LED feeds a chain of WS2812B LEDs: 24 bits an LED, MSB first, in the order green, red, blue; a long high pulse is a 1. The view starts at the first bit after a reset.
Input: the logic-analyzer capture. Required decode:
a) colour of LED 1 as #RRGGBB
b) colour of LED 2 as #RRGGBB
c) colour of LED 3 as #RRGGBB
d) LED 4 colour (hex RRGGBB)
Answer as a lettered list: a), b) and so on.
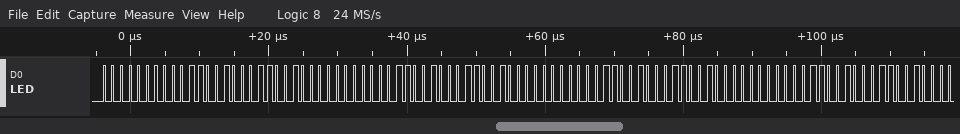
a) #320032
b) #320032
c) #320032
d) #320032
